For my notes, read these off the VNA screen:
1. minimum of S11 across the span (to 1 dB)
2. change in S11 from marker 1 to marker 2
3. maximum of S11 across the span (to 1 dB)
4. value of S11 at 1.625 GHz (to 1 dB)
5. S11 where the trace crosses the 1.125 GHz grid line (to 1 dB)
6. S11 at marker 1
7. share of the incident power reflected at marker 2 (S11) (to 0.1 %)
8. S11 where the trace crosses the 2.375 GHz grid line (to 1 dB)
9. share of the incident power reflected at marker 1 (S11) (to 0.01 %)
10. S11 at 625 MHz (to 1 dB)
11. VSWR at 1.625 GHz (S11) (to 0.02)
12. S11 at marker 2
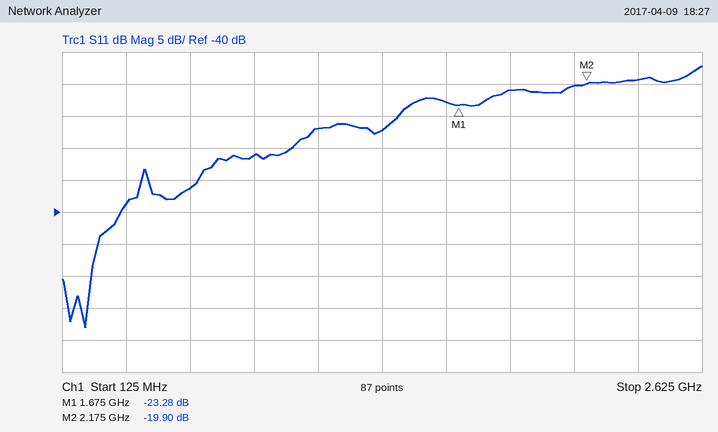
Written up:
-58 dB
3.38 dB
-17 dB
-23 dB
-27 dB
-23.28 dB
1.0 %
-19 dB
0.47 %
-36 dB
1.16
-19.90 dB
